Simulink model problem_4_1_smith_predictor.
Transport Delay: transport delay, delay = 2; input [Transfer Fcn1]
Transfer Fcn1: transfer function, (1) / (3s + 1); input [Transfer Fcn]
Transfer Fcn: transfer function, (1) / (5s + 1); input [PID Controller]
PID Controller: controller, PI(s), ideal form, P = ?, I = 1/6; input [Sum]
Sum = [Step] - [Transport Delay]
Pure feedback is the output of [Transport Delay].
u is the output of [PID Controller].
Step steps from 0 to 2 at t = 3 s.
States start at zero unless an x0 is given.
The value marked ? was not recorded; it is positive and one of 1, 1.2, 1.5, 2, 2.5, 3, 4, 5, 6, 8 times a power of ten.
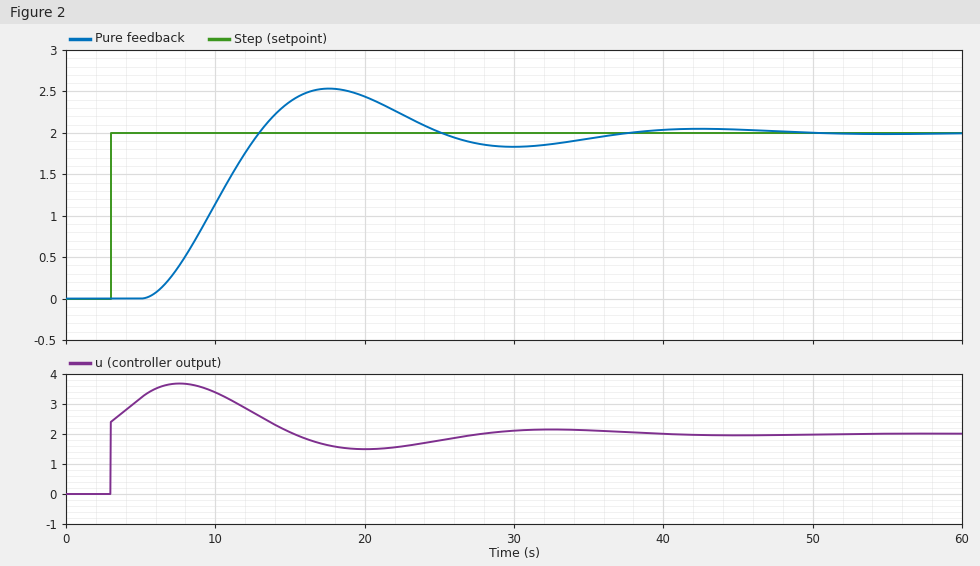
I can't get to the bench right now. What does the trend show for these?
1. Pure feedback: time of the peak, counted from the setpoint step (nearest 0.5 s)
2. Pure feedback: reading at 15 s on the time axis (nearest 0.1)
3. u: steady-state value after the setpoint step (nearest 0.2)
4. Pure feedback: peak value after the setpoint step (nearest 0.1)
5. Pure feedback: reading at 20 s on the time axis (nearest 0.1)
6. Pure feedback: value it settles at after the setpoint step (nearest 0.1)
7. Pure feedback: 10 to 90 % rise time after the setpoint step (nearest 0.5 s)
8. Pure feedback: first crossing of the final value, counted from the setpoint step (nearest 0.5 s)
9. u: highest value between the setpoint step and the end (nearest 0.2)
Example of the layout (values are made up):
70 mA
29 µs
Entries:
14.5 s
2.4
2.0
2.5
2.4
2.0
5.5 s
10.0 s
3.6
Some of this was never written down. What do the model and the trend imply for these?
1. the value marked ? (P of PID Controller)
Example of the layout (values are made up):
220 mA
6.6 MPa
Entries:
1.2
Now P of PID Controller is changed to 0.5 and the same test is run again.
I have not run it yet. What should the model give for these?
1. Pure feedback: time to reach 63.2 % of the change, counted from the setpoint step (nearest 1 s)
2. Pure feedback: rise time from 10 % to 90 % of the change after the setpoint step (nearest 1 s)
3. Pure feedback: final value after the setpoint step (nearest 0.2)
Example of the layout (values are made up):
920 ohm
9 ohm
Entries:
13 s
16 s
2.0
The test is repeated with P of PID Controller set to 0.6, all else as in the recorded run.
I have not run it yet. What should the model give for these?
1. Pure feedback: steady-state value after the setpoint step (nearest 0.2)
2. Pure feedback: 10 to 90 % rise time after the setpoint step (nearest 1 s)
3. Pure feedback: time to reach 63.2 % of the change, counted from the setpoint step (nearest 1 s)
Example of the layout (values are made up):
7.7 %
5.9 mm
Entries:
2.0
12 s
11 s
